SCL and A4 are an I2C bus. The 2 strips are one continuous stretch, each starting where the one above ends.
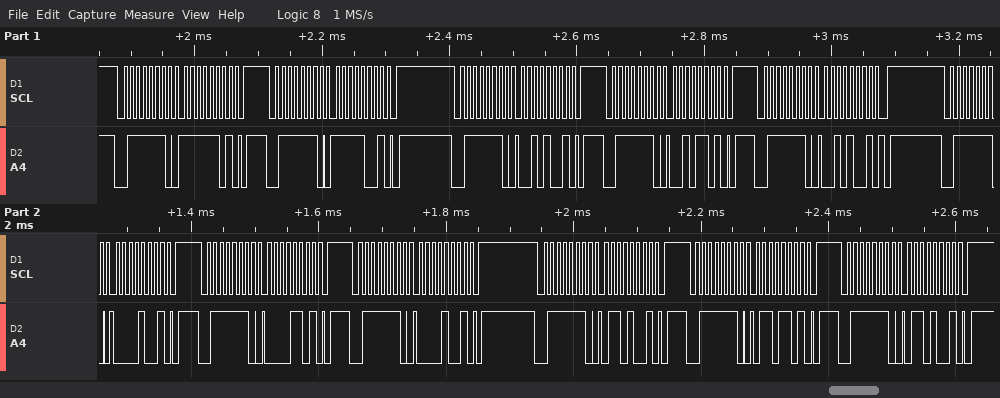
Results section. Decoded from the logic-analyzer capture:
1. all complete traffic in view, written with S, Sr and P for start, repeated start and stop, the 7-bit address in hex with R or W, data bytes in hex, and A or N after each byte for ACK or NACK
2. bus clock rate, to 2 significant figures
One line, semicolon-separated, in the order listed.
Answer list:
S 3FW A FD A P S 3FW A F9 A P S 3FW A 29 A P S 3FW A 2D A P S 3FW A 29 A P S 3FW A 09 A P S 3FW A 0D A P S 3FW A 09 A P S 3FW A 69 A P S 3FW A 6D A P S 3FW A 69 A P; 100 kHz
